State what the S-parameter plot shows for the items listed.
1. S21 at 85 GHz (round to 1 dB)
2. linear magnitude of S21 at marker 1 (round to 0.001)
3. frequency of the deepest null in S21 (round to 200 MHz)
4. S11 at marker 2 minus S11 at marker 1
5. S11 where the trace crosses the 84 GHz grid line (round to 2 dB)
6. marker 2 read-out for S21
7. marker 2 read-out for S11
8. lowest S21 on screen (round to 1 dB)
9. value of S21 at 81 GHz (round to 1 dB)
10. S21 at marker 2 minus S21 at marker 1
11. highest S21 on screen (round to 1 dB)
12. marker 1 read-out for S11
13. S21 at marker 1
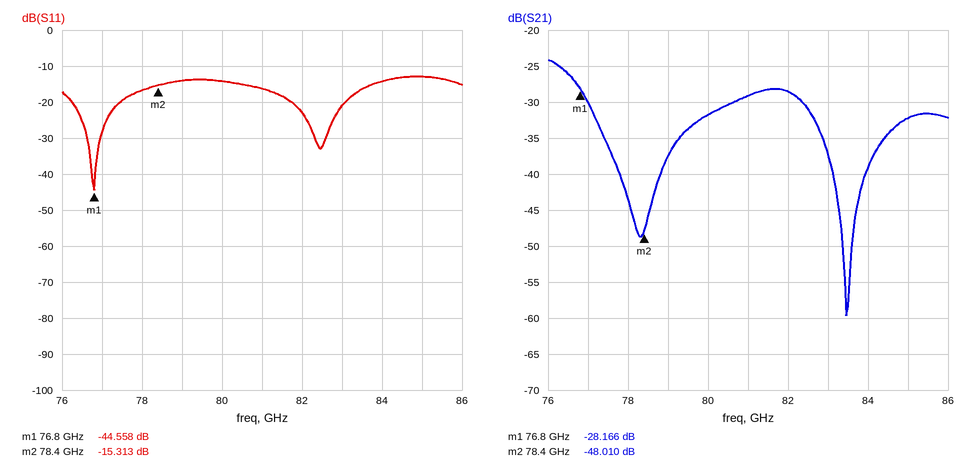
-32 dB
0.039
83.4 GHz
29.245 dB
-14 dB
-48.010 dB
-15.313 dB
-60 dB
-29 dB
-19.844 dB
-24 dB
-44.558 dB
-28.166 dB
